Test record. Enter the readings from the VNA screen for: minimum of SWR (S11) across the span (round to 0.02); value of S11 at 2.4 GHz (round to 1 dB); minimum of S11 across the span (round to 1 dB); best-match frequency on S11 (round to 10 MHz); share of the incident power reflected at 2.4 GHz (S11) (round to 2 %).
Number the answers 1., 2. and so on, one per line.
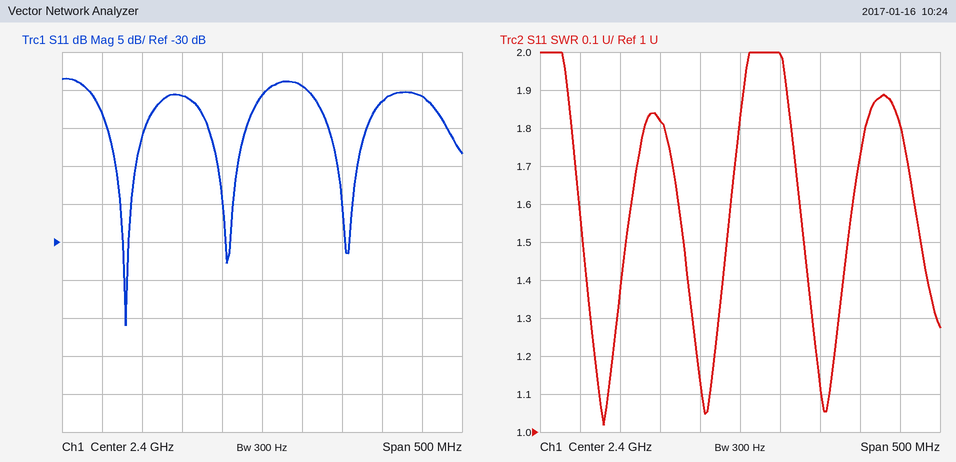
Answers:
1. 1.02
2. -11 dB
3. -41 dB
4. 2.23 GHz
5. 8 %
